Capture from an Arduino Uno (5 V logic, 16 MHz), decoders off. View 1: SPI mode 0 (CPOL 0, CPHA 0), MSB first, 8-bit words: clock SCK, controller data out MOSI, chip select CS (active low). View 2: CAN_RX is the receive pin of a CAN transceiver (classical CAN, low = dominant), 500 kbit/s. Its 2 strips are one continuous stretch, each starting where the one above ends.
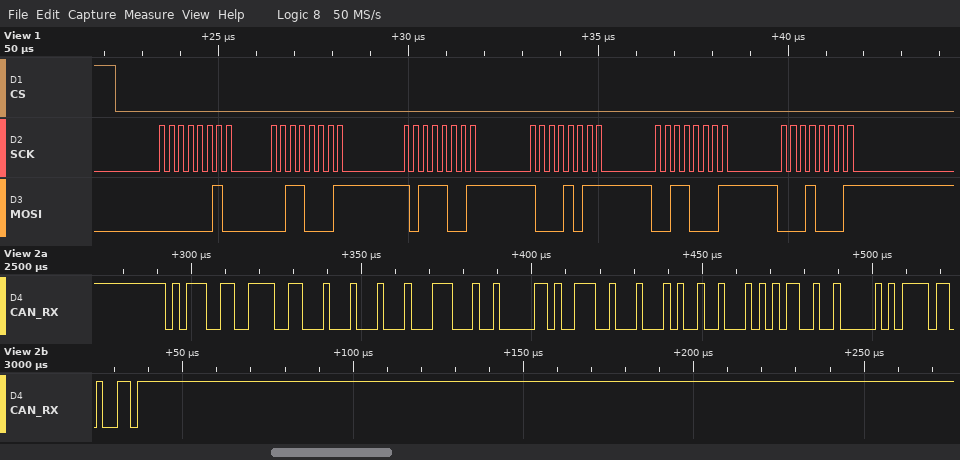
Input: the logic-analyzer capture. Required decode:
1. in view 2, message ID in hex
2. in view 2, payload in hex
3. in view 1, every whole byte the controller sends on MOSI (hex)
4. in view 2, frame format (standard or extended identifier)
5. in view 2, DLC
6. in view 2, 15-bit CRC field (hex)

0x17333111
E2 41 4E 44 52 45 59 20
02 31 B9 8B 31 11
extended
8
0x2F69
